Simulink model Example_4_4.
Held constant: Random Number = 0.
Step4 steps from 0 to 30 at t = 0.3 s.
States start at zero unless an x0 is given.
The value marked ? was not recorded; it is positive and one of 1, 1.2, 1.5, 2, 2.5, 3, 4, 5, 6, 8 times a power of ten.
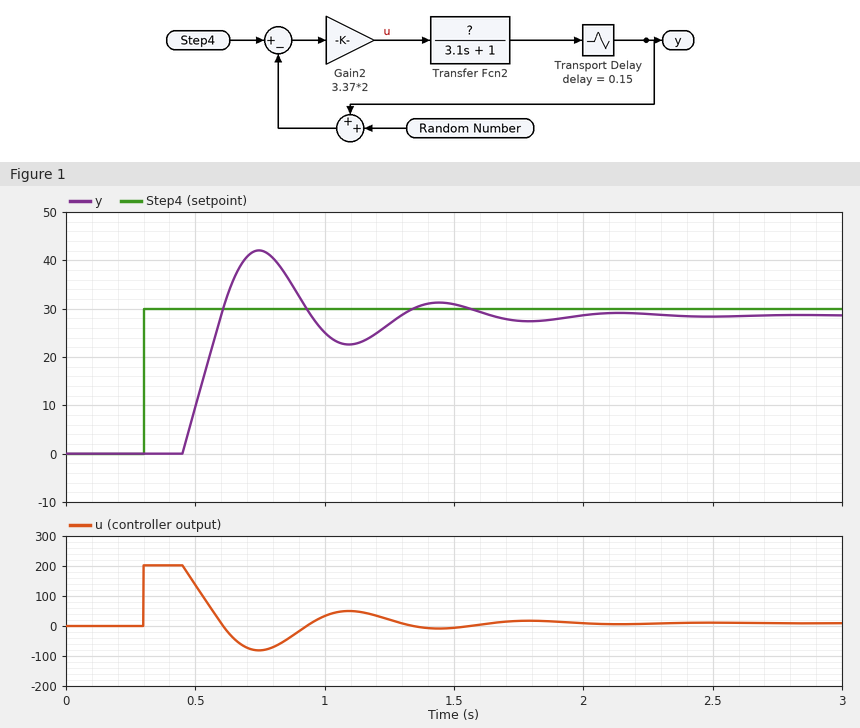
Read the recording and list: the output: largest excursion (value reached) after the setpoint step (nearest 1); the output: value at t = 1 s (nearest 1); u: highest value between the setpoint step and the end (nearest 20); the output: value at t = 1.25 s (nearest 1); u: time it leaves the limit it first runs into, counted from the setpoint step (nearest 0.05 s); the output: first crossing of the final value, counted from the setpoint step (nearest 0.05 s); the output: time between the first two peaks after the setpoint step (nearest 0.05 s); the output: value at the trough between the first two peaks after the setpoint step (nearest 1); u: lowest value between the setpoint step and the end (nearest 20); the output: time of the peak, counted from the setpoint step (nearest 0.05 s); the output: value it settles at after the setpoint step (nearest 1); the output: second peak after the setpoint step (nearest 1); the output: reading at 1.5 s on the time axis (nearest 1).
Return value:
42
25
200
27
0.15 s
0.30 s
0.70 s
23
-80
0.45 s
29
31
31
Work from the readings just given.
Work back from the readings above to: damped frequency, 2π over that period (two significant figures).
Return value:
9.0 rad/s
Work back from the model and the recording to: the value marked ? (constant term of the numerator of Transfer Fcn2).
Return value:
3
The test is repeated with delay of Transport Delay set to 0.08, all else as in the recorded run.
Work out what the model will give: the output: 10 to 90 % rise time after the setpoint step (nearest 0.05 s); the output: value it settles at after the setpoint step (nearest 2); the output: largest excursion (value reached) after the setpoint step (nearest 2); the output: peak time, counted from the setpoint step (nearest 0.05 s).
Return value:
0.15 s
28
30
0.35 s
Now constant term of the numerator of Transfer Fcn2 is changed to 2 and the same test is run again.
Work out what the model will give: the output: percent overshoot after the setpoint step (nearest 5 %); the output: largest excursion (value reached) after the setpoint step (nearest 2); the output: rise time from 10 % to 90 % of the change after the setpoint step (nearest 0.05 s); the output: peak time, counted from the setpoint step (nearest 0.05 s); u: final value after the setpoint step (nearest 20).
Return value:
15 %
32
0.20 s
0.55 s
20
